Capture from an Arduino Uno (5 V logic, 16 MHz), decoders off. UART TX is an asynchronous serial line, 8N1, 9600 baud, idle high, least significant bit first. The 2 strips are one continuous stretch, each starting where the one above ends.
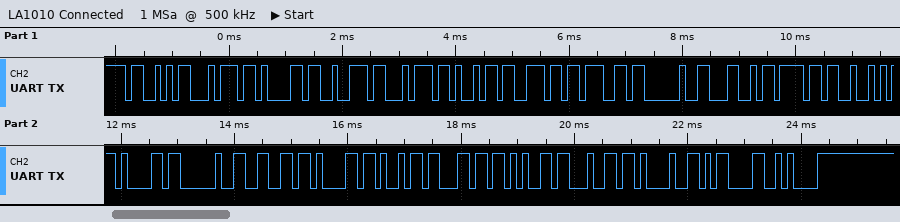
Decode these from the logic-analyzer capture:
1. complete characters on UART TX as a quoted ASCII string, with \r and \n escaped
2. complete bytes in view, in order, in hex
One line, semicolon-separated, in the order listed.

"Starting LoRa failed!\r\n"; 53 74 61 72 74 69 6E 67 20 4C 6F 52 61 20 66 61 69 6C 65 64 21 0D 0A
